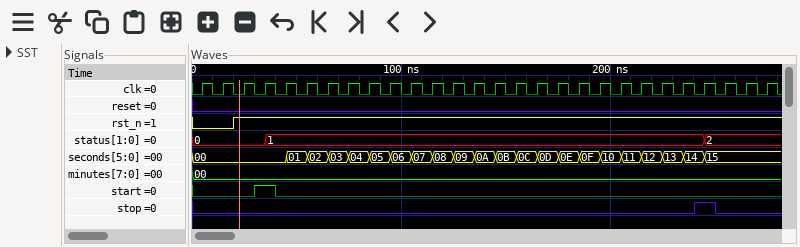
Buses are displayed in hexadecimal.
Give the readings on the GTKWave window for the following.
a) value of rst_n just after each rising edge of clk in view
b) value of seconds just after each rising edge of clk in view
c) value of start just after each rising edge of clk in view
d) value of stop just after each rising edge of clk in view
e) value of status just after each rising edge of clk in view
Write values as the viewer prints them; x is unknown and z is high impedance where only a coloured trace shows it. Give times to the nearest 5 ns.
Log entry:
0 0 1 1 1 1 1 1 1 1 1 1 1 1 1 1 1 1 1 1 1 1 1 1 1 1 1 1
00, 00, 00, 00, 01, 02, 03, 04, 05, 06, 07, 08, 09, 0A, 0B, 0C, 0D, 0E, 0F, 10, 11, 12, 13, 14, 15, 15, 15, 15
0 0 0 1 0 0 0 0 0 0 0 0 0 0 0 0 0 0 0 0 0 0 0 0 0 0 0 0
0 0 0 0 0 0 0 0 0 0 0 0 0 0 0 0 0 0 0 0 0 0 0 0 1 0 0 0
0, 0, 0, 1, 1, 1, 1, 1, 1, 1, 1, 1, 1, 1, 1, 1, 1, 1, 1, 1, 1, 1, 1, 1, 2, 2, 2, 2
